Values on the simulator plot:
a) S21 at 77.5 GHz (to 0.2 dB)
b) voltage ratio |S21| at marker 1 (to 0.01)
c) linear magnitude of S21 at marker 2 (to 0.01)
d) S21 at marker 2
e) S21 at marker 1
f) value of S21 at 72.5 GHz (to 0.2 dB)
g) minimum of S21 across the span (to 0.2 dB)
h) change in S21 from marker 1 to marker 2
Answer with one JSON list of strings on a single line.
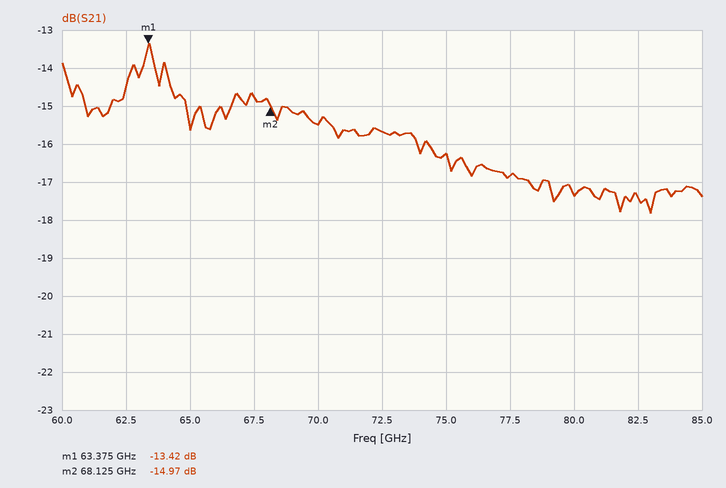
["-16.8 dB", "0.21", "0.18", "-14.97 dB", "-13.42 dB", "-15.6 dB", "-17.8 dB", "-1.55 dB"]
